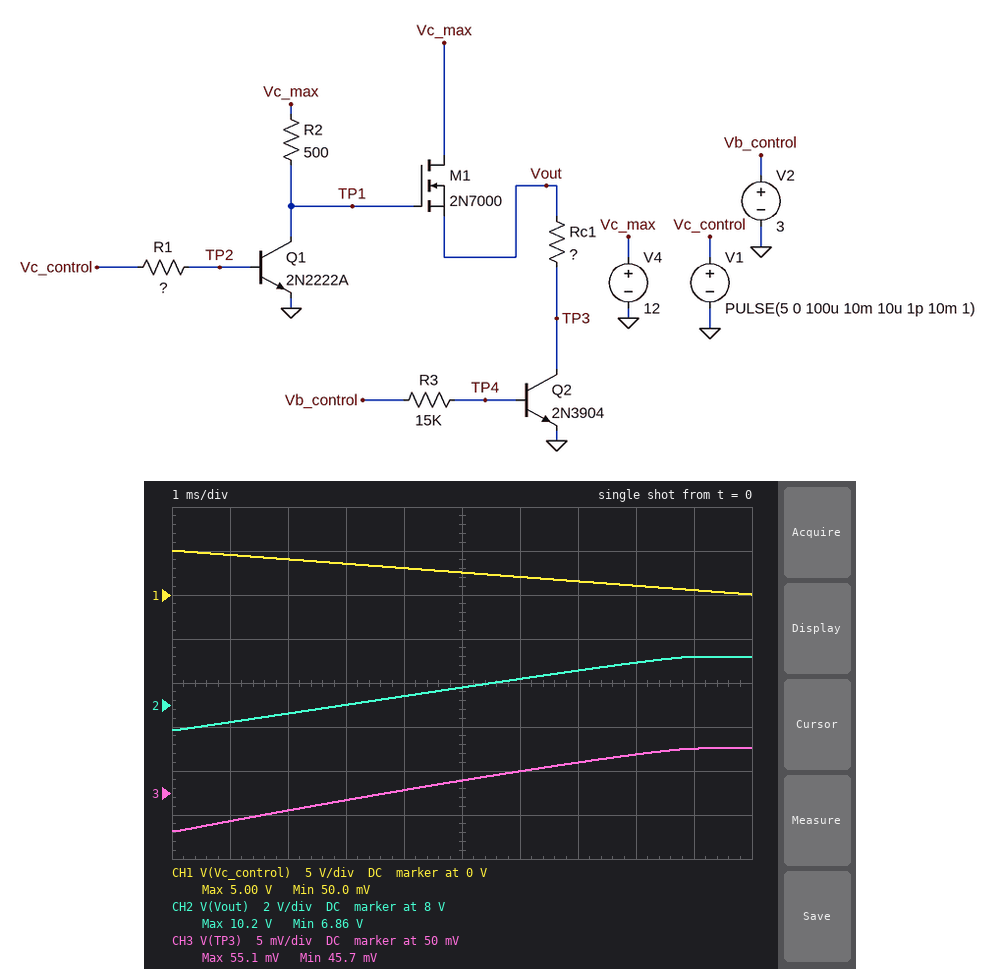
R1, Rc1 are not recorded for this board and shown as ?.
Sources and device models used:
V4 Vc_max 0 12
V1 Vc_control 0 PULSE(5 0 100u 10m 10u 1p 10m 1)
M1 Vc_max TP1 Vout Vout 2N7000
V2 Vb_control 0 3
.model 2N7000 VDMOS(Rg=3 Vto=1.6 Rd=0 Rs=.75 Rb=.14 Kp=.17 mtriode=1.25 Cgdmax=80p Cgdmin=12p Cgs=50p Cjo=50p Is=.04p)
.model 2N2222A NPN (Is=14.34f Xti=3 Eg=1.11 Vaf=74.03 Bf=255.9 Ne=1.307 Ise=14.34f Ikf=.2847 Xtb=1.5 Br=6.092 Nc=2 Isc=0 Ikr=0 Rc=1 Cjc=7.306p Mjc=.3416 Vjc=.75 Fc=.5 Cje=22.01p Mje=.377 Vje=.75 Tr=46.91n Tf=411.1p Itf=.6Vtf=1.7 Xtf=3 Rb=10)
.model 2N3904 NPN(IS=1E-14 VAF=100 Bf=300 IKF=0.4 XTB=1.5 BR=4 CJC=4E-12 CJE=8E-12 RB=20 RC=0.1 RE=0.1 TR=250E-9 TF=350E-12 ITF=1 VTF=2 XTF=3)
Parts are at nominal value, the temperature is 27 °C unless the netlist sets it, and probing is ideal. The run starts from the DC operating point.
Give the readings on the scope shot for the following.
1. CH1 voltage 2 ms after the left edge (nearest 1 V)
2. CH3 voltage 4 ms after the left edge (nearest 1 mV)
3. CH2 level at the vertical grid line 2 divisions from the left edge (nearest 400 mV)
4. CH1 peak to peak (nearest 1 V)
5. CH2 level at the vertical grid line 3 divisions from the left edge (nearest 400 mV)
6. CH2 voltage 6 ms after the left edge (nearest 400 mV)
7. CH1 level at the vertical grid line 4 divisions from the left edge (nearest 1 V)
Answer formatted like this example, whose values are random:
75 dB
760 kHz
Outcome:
4 V
50 mV
7.6 V
5 V
8.0 V
9.2 V
3 V
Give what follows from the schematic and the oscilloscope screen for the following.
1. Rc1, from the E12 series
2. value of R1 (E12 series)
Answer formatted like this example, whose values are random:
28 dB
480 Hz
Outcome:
2.7 kΩ
120 kΩ
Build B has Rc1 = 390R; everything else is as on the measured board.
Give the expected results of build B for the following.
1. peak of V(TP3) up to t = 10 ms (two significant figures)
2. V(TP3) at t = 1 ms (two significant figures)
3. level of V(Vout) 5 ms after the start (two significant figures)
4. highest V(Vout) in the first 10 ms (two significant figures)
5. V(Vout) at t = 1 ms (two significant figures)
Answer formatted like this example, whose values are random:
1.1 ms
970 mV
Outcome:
130 mV
110 mV
8.5 V
9.8 V
6.9 V
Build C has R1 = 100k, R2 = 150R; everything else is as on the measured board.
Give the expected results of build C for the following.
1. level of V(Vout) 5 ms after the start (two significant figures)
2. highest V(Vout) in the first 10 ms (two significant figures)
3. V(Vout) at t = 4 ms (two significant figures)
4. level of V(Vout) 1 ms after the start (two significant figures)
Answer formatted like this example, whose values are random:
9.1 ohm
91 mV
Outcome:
9.7 V
10 V
9.5 V
9.1 V
